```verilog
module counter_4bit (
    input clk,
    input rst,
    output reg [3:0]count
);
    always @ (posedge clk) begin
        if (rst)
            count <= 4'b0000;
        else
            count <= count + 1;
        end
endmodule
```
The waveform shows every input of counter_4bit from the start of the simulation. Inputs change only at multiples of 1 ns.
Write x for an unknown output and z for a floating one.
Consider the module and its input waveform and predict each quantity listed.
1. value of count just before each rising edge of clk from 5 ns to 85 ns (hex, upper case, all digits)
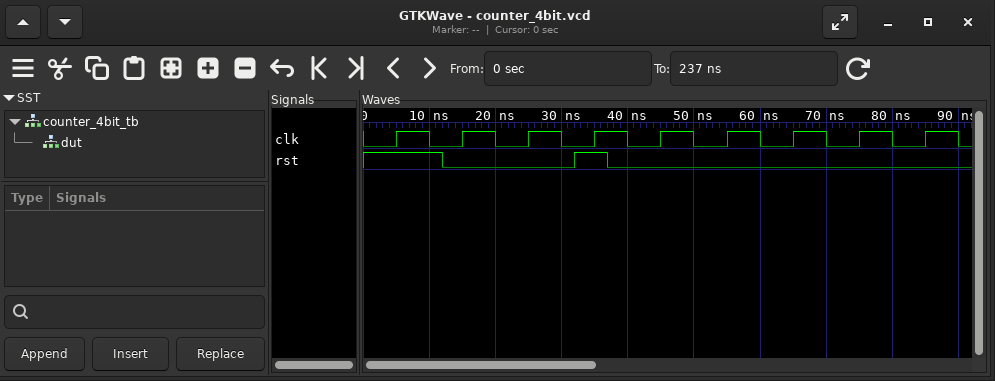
x, 0, 1, 2, 0, 1, 2, 3, 4
